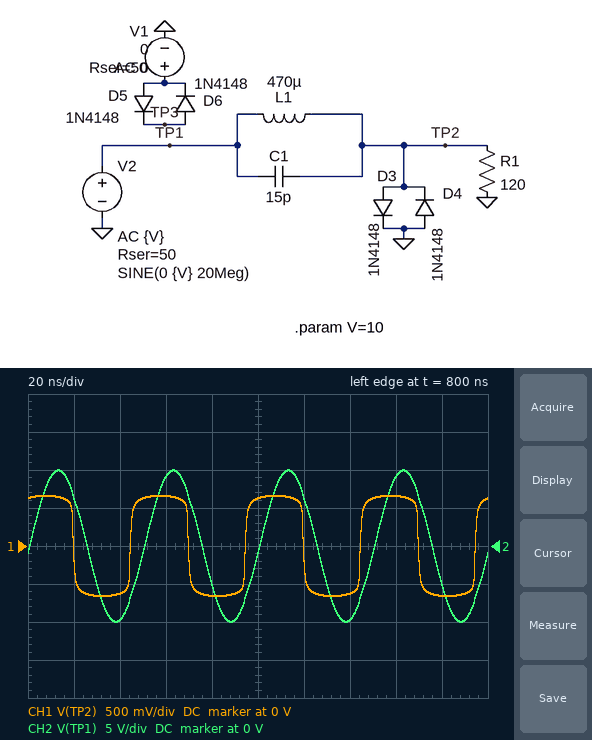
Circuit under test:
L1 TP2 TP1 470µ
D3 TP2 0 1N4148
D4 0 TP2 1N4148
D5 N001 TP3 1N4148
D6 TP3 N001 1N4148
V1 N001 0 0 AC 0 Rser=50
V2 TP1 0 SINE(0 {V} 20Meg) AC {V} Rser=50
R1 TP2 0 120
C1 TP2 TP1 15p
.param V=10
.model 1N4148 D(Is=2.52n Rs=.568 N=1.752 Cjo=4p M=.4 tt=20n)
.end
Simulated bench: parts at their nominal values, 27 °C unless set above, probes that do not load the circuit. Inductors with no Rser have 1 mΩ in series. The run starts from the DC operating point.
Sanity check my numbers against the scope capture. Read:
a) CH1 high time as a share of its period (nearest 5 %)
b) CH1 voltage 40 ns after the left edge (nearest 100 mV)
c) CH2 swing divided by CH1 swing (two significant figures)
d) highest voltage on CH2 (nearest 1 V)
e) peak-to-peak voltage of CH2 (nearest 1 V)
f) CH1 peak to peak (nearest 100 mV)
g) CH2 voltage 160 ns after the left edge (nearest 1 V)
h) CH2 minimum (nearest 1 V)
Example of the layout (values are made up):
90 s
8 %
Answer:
50 %
-600 mV
15
10 V
20 V
1.3 V
9 V
-10 V
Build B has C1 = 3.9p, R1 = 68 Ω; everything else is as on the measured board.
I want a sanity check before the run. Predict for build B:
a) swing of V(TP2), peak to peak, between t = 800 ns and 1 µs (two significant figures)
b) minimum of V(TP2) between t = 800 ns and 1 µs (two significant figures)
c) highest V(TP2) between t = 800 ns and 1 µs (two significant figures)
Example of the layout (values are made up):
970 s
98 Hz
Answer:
640 mV
-310 mV
330 mV
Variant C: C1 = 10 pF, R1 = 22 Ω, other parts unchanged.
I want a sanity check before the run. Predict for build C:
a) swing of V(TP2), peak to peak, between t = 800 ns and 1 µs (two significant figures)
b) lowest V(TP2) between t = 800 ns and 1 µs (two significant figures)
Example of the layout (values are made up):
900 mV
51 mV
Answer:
540 mV
-270 mV
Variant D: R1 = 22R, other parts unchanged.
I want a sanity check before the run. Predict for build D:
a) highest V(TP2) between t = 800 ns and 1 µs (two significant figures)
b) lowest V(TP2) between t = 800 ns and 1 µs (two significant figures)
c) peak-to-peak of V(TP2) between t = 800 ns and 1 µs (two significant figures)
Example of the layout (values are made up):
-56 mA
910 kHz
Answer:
410 mV
-400 mV
810 mV
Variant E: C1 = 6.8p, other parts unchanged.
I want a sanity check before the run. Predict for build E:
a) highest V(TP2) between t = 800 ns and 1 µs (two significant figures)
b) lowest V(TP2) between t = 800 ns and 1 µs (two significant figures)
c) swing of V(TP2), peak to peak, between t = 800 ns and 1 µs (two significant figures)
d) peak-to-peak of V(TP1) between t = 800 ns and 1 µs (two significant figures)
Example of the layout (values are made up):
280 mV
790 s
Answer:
600 mV
-590 mV
1.2 V
20 V
